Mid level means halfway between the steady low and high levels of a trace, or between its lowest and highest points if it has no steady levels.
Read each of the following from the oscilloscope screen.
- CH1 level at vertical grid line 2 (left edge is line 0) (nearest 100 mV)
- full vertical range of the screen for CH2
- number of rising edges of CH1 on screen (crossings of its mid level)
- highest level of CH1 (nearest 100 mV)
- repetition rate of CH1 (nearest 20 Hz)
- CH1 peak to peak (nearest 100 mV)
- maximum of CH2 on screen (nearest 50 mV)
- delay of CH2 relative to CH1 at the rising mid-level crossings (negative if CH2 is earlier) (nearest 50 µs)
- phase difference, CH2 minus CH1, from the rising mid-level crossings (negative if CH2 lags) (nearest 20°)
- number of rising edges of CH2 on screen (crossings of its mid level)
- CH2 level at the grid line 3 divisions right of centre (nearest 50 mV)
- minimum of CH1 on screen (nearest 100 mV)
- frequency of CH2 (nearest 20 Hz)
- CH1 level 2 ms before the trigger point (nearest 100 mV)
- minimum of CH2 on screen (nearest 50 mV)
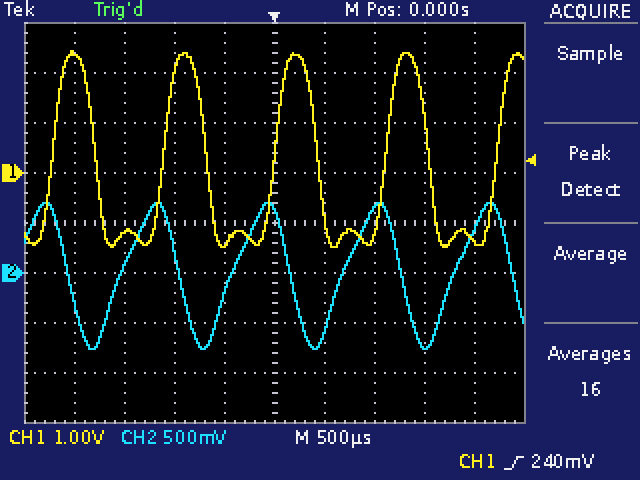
-1.2 V
4 V
5
2.4 V
900 Hz
3.9 V
700 mV
-450 µs
+140°
4
-750 mV
-1.5 V
900 Hz
2.4 V
-750 mV
